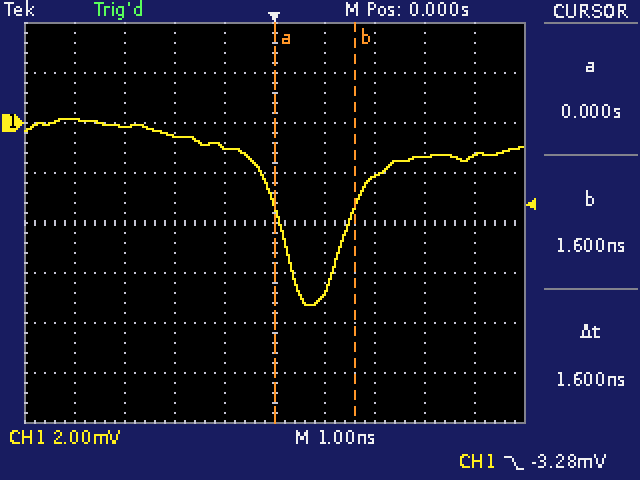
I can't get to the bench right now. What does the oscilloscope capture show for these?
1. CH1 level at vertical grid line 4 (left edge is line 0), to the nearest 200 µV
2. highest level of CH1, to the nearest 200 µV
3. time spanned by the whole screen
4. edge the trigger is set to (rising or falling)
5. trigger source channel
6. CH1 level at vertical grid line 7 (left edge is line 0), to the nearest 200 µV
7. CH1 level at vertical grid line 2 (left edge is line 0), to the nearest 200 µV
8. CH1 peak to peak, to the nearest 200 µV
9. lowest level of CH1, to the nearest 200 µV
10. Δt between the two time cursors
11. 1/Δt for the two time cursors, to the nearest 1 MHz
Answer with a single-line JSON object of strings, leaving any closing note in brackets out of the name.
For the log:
{"CH1 level at vertical grid line 4 (left edge is line 0), to the nearest 200 µV": "-1.0 mV", "highest level of CH1, to the nearest 200 µV": "200 µV", "time spanned by the whole screen": "10 ns", "edge the trigger is set to": "falling", "trigger source channel": "CH1", "CH1 level at vertical grid line 7 (left edge is line 0), to the nearest 200 µV": "-2.2 mV", "CH1 level at vertical grid line 2 (left edge is line 0), to the nearest 200 µV": "-200 µV", "CH1 peak to peak, to the nearest 200 µV": "7.4 mV", "lowest level of CH1, to the nearest 200 µV": "-7.2 mV", "Δt between the two time cursors": "1.6 ns", "1/Δt for the two time cursors, to the nearest 1 MHz": "625 MHz"}
